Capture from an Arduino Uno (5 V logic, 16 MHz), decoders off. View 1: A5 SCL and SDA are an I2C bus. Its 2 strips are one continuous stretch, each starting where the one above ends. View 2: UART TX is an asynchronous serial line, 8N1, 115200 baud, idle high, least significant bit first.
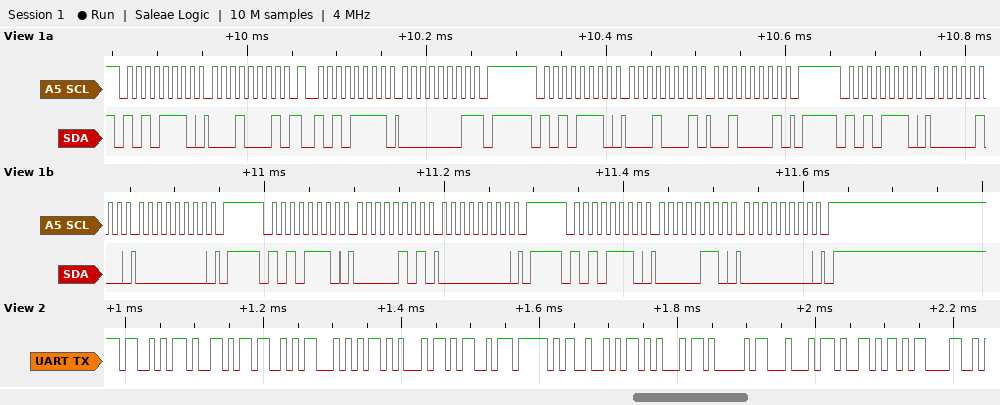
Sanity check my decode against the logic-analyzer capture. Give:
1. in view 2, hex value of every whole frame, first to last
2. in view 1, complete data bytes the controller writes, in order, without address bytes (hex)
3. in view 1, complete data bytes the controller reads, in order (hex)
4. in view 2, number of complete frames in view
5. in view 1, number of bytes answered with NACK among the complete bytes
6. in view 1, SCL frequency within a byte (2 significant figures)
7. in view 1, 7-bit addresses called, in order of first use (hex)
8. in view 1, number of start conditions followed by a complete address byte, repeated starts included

0x53 0x59 0x53 0x54 0x45 0x4D 0x5F 0x52 0x45 0x41 0x44 0x59 0x0D
11 11 21 04 00 05 00 06 00
01
13
1
100 kHz
0x57
6
